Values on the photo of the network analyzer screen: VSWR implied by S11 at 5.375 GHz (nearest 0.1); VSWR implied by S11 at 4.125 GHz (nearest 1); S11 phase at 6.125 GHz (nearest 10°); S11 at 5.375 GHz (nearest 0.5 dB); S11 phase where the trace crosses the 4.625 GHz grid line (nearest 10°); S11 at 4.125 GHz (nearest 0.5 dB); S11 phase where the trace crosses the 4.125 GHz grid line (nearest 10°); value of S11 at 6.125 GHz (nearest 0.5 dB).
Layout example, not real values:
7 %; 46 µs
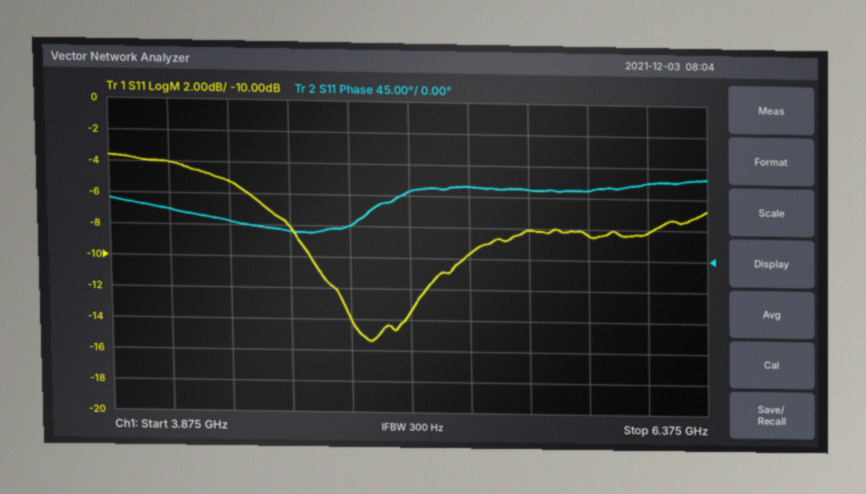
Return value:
2.0; 4; 110°; -9.5 dB; 40°; -4.0 dB; 70°; -8.0 dB
